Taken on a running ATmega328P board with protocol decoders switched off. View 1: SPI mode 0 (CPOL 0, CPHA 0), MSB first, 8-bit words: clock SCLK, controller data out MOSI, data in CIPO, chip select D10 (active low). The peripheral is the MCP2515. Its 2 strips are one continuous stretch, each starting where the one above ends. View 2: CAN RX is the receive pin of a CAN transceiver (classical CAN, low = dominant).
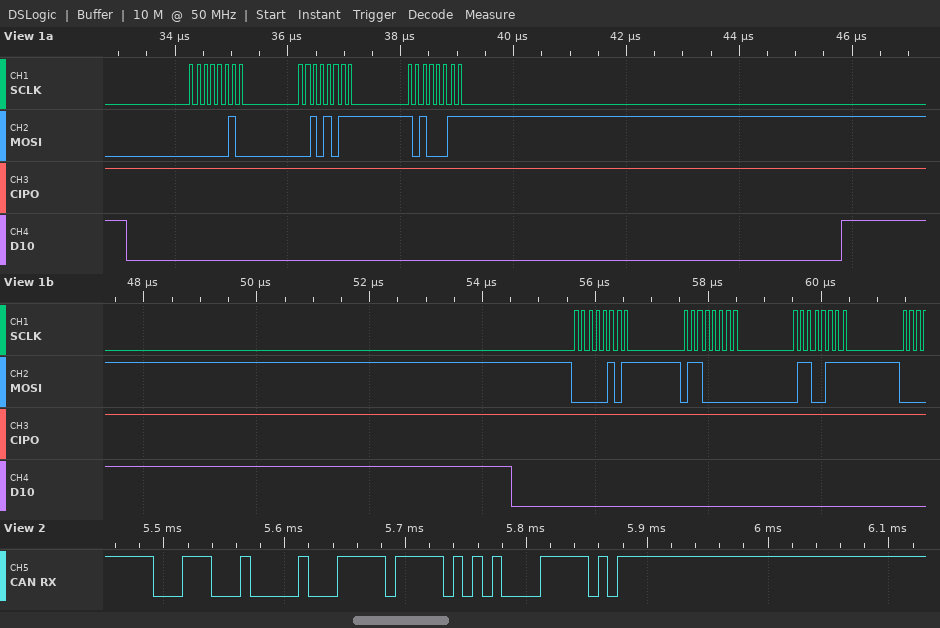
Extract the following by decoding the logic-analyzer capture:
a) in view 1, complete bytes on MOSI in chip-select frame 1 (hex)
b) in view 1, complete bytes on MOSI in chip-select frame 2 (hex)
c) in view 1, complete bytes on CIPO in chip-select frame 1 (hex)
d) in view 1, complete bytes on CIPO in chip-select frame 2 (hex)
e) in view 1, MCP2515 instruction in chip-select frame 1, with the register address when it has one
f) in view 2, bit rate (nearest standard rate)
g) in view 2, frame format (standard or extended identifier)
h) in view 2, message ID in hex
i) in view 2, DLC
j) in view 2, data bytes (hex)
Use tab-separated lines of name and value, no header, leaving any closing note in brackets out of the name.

in view 1, complete bytes on MOSI in chip-select frame 1	0x02 0x2B 0xA3
in view 1, complete bytes on MOSI in chip-select frame 2	0x05 0x60 0x67
in view 1, complete bytes on CIPO in chip-select frame 1	0xFF 0xFF 0xFF
in view 1, complete bytes on CIPO in chip-select frame 2	0xFF 0xFF 0xFF
in view 1, MCP2515 instruction in chip-select frame 1, with the register address when it has one	WRITE 0x2B
in view 2, bit rate	125 kbit/s
in view 2, frame format	standard
in view 2, message ID in hex	0x1C4
in view 2, DLC	1
in view 2, data bytes	FF
